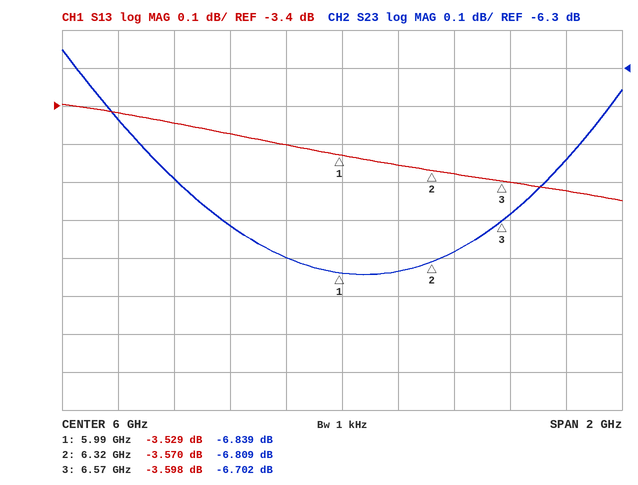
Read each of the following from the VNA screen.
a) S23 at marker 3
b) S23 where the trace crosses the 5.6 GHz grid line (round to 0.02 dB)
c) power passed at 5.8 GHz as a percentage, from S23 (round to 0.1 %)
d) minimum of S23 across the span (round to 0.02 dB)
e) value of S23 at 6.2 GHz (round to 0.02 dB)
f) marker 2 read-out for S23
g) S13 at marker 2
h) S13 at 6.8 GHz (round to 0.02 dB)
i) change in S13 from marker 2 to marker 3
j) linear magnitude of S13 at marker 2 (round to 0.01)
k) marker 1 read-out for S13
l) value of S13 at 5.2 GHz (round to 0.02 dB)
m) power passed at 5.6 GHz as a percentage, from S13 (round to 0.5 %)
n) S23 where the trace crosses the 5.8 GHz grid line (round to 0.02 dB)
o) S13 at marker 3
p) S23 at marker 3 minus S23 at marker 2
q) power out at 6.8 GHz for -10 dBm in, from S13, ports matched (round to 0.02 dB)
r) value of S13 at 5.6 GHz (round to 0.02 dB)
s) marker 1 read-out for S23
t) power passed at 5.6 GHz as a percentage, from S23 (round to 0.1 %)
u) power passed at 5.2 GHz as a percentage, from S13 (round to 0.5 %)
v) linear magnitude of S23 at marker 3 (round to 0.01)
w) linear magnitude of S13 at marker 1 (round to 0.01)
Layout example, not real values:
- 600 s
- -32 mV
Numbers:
- -6.702 dB
- -6.72 dB
- 20.9 %
- -6.84 dB
- -6.84 dB
- -6.809 dB
- -3.570 dB
- -3.62 dB
- -0.028 dB
- 0.66
- -3.529 dB
- -3.42 dB
- 45.0 %
- -6.80 dB
- -3.598 dB
- 0.107 dB
- -13.62 dBm
- -3.48 dB
- -6.839 dB
- 21.3 %
- 45.5 %
- 0.46
- 0.67
